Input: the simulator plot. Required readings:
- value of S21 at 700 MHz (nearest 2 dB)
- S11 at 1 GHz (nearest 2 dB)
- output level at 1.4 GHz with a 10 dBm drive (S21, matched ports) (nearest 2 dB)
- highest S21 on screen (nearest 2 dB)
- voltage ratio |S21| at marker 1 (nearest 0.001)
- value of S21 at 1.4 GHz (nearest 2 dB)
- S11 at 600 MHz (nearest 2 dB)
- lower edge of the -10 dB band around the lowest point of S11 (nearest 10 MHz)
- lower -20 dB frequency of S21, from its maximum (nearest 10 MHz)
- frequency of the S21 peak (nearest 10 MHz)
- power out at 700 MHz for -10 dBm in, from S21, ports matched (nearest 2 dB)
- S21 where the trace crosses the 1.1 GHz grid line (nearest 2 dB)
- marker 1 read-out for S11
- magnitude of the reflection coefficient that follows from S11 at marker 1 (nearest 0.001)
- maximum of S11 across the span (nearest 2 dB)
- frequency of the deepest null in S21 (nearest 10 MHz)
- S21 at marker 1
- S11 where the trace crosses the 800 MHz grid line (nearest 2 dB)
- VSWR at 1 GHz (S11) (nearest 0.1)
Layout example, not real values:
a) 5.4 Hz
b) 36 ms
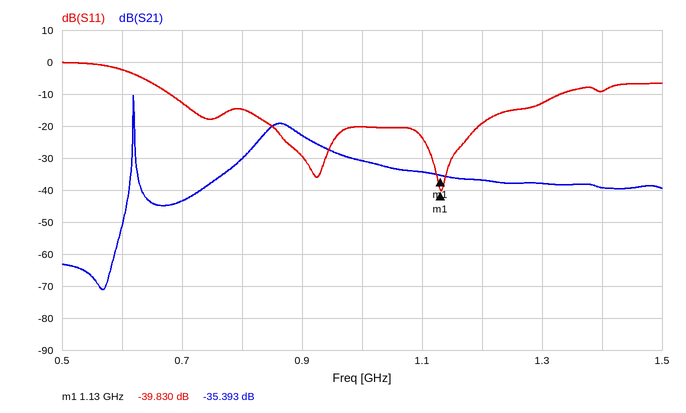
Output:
a) -44 dB
b) -20 dB
c) -30 dBm
d) -10 dB
e) 0.017
f) -40 dB
g) -2 dB
h) 680 MHz
i) 620 MHz
j) 620 MHz
k) -54 dBm
l) -34 dB
m) -39.830 dB
n) 0.010
o) 0 dB
p) 570 MHz
q) -35.393 dB
r) -14 dB
s) 1.2
